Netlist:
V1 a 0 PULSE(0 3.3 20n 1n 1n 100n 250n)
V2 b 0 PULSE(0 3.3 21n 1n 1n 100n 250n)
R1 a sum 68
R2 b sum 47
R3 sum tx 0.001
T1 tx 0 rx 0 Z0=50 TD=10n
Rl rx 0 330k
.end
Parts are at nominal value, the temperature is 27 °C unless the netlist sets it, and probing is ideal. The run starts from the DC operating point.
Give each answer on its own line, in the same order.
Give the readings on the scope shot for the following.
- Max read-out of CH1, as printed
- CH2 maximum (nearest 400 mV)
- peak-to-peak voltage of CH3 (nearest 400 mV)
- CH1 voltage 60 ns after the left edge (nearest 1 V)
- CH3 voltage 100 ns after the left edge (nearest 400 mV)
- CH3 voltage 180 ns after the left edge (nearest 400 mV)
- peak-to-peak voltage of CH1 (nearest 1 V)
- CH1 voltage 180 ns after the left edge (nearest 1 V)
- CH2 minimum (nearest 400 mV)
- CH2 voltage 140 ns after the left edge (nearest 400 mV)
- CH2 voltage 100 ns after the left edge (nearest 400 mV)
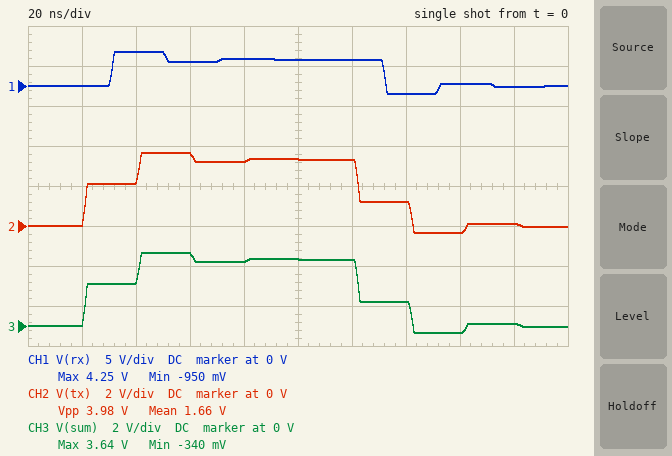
4.25 V
3.6 V
4.0 V
3 V
3.2 V
0 V
5 V
0 V
-400 mV
1.2 V
3.2 V
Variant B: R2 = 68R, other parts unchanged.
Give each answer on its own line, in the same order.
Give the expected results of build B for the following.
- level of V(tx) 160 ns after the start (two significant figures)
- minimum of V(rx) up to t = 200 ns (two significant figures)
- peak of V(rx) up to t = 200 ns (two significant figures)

-250 mV
-630 mV
3.9 V
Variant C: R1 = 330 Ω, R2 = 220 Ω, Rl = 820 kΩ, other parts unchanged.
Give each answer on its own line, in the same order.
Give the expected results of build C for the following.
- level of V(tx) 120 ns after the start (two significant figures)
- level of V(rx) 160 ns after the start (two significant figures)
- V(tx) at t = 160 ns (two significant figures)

3.2 V
660 mV
1.1 V
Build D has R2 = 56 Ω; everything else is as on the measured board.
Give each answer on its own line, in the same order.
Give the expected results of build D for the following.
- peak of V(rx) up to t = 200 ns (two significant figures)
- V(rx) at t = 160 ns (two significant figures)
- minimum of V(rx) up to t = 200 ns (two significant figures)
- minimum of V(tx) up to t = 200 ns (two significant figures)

4.1 V
190 mV
-790 mV
-300 mV
